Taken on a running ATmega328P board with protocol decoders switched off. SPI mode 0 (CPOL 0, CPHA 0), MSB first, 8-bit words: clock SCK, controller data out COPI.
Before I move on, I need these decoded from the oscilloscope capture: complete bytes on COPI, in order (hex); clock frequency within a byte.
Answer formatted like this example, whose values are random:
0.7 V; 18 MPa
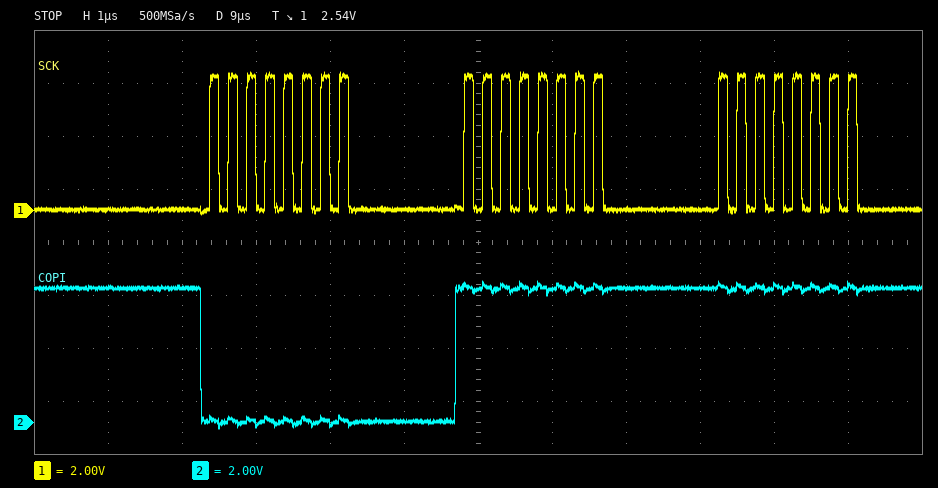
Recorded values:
00 FF FF; 4 MHz
